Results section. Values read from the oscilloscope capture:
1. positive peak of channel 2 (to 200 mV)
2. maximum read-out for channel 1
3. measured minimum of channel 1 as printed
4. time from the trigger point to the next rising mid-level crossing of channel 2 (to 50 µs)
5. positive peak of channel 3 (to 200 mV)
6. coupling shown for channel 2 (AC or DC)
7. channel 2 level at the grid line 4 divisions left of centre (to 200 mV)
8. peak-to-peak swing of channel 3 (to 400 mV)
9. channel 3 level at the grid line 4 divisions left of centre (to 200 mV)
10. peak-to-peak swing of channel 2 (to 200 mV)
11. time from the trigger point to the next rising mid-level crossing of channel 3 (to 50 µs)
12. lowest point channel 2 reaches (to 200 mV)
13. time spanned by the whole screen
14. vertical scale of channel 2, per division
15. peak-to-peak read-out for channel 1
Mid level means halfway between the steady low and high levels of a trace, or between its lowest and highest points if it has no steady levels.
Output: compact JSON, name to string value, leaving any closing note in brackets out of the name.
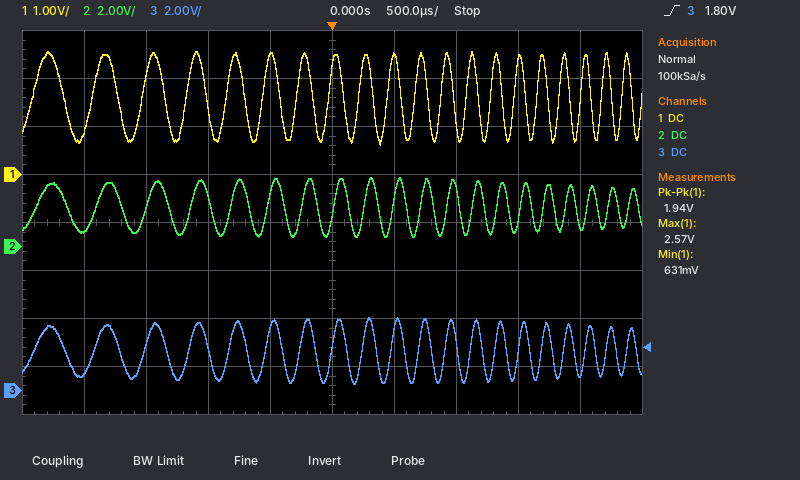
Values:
{"positive peak of channel 2": "2.8 V", "maximum read-out for channel 1": "2.57 V", "measured minimum of channel 1 as printed": "631 mV", "time from the trigger point to the next rising mid-level crossing of channel 2": "250 µs", "positive peak of channel 3": "3.0 V", "coupling shown for channel 2": "DC", "channel 2 level at the grid line 4 divisions left of centre": "600 mV", "peak-to-peak swing of channel 3": "2.8 V", "channel 3 level at the grid line 4 divisions left of centre": "800 mV", "peak-to-peak swing of channel 2": "2.4 V", "time from the trigger point to the next rising mid-level crossing of channel 3": "250 µs", "lowest point channel 2 reaches": "400 mV", "time spanned by the whole screen": "5 ms", "vertical scale of channel 2, per division": "2 V", "peak-to-peak read-out for channel 1": "1.94 V"}
